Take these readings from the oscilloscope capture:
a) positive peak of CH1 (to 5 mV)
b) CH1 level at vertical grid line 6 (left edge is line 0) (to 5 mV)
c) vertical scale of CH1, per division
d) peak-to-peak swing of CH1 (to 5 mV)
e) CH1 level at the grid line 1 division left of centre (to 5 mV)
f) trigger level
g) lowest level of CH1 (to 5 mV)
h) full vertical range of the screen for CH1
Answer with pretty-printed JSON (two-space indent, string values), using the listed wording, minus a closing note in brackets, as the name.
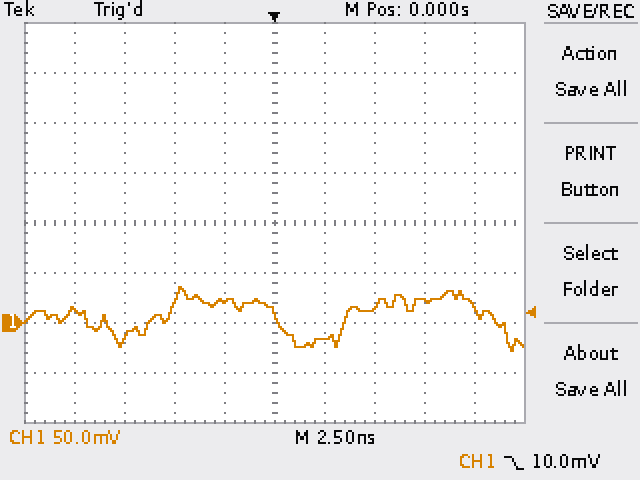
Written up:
{
  "positive peak of CH1": "35 mV",
  "CH1 level at vertical grid line 6 (left edge is line 0)": "-15 mV",
  "vertical scale of CH1, per division": "50 mV",
  "peak-to-peak swing of CH1": "65 mV",
  "CH1 level at the grid line 1 division left of centre": "20 mV",
  "trigger level": "10.0 mV",
  "lowest level of CH1": "-30 mV",
  "full vertical range of the screen for CH1": "400 mV"
}
